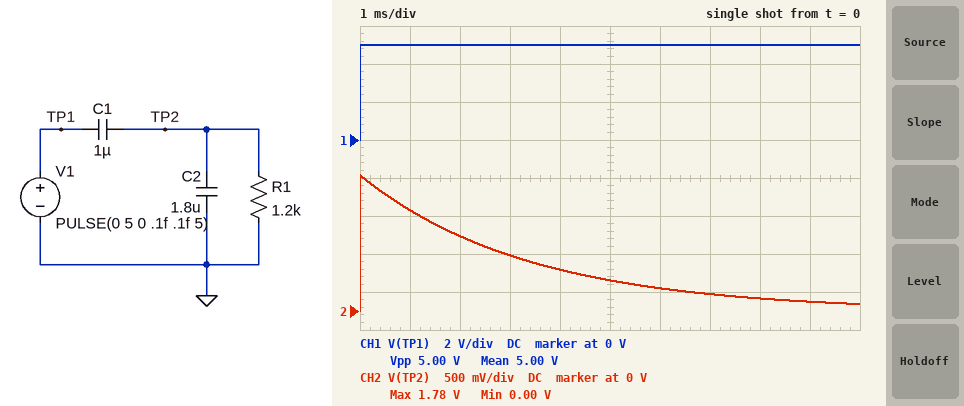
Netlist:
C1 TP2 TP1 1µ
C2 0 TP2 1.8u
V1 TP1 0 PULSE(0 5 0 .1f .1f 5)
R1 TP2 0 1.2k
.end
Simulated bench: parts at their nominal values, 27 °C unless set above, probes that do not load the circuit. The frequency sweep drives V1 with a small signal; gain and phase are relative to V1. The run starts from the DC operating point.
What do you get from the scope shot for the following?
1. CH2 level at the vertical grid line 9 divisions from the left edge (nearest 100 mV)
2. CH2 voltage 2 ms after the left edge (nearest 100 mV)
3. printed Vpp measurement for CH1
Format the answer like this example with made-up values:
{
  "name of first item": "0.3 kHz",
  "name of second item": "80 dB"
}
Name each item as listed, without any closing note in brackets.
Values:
{
  "CH2 level at the vertical grid line 9 divisions from the left edge": "100 mV",
  "CH2 voltage 2 ms after the left edge": "1.0 V",
  "printed Vpp measurement for CH1": "5.00 V"
}
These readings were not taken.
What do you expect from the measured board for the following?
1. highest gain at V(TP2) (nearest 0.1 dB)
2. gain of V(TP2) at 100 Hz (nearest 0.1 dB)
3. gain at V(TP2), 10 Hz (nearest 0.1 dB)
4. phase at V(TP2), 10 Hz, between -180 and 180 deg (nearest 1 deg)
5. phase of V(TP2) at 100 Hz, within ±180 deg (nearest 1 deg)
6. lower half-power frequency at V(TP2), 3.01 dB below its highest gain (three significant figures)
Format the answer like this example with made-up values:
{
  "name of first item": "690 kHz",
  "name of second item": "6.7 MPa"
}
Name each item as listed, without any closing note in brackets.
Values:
{
  "highest gain at V(TP2)": "-8.9 dB",
  "gain of V(TP2) at 100 Hz": "-9.8 dB",
  "gain at V(TP2), 10 Hz": "-22.6 dB",
  "phase at V(TP2), 10 Hz, between -180 and 180 deg": "78 deg",
  "phase of V(TP2) at 100 Hz, within ±180 deg": "25 deg",
  "lower half-power frequency at V(TP2), 3.01 dB below its highest gain": "47.4 Hz"
}
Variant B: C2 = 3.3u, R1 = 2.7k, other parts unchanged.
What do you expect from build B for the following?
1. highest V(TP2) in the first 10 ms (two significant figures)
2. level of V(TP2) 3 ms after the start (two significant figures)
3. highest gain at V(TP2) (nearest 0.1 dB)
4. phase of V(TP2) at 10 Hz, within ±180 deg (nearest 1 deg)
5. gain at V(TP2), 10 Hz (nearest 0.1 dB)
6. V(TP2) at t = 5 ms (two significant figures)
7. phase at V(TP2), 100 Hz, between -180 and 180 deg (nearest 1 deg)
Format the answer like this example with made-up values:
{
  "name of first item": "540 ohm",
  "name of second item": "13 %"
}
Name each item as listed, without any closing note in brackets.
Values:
{
  "highest V(TP2) in the first 10 ms": "1.2 V",
  "level of V(TP2) 3 ms after the start": "900 mV",
  "highest gain at V(TP2)": "-12.7 dB",
  "phase of V(TP2) at 10 Hz, within ±180 deg": "54 deg",
  "gain at V(TP2), 10 Hz": "-17.3 dB",
  "V(TP2) at t = 5 ms": "760 mV",
  "phase at V(TP2), 100 Hz, between -180 and 180 deg": "8 deg"
}
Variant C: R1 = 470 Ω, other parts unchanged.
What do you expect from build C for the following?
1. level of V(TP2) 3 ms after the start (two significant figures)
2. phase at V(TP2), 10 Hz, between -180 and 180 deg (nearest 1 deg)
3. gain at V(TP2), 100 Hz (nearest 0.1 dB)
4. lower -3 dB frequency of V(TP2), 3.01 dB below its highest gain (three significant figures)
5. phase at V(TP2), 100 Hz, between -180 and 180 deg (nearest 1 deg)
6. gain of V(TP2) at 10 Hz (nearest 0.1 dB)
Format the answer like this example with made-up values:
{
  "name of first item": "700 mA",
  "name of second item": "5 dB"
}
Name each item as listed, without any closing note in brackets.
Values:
{
  "level of V(TP2) 3 ms after the start": "180 mV",
  "phase at V(TP2), 10 Hz, between -180 and 180 deg": "85 deg",
  "gain at V(TP2), 100 Hz": "-12.9 dB",
  "lower -3 dB frequency of V(TP2), 3.01 dB below its highest gain": "121 Hz",
  "phase at V(TP2), 100 Hz, between -180 and 180 deg": "50 deg",
  "gain of V(TP2) at 10 Hz": "-30.6 dB"
}
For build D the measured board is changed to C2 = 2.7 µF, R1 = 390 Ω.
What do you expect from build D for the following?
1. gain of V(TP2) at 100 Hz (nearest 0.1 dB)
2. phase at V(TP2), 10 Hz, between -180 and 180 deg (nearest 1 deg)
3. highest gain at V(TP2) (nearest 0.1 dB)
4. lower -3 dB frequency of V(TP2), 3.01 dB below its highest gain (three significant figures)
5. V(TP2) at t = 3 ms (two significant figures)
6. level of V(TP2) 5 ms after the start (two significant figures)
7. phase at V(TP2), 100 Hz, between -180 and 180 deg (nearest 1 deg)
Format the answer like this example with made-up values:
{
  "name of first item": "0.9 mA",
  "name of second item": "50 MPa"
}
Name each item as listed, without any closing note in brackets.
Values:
{
  "gain of V(TP2) at 100 Hz": "-14.8 dB",
  "phase at V(TP2), 10 Hz, between -180 and 180 deg": "85 deg",
  "highest gain at V(TP2)": "-11.4 dB",
  "lower -3 dB frequency of V(TP2), 3.01 dB below its highest gain": "110 Hz",
  "V(TP2) at t = 3 ms": "170 mV",
  "level of V(TP2) 5 ms after the start": "42 mV",
  "phase at V(TP2), 100 Hz, between -180 and 180 deg": "48 deg"
}
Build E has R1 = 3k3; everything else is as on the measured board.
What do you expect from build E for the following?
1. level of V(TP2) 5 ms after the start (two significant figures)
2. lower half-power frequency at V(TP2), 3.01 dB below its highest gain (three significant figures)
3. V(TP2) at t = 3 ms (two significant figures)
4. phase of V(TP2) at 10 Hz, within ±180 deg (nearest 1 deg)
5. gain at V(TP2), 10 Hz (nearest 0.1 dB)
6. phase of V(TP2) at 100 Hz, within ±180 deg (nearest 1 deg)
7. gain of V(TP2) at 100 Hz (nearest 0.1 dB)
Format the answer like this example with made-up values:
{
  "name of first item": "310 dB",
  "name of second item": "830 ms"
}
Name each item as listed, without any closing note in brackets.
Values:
{
  "level of V(TP2) 5 ms after the start": "1.0 V",
  "lower half-power frequency at V(TP2), 3.01 dB below its highest gain": "17.2 Hz",
  "V(TP2) at t = 3 ms": "1.3 V",
  "phase of V(TP2) at 10 Hz, within ±180 deg": "60 deg",
  "gain at V(TP2), 10 Hz": "-14.9 dB",
  "phase of V(TP2) at 100 Hz, within ±180 deg": "10 deg",
  "gain of V(TP2) at 100 Hz": "-9.1 dB"
}
